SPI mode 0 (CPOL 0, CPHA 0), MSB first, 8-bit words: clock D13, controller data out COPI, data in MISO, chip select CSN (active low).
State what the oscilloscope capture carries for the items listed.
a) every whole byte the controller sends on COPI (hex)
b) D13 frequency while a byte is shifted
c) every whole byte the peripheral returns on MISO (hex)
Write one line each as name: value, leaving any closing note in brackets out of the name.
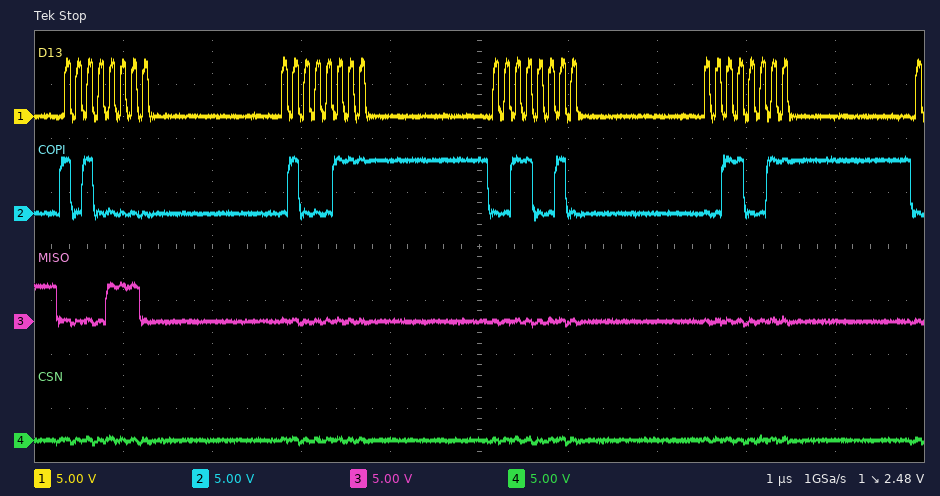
every whole byte the controller sends on COPI: A0 47 32 33
D13 frequency while a byte is shifted: 8 MHz
every whole byte the peripheral returns on MISO: 0E 00 00 00
